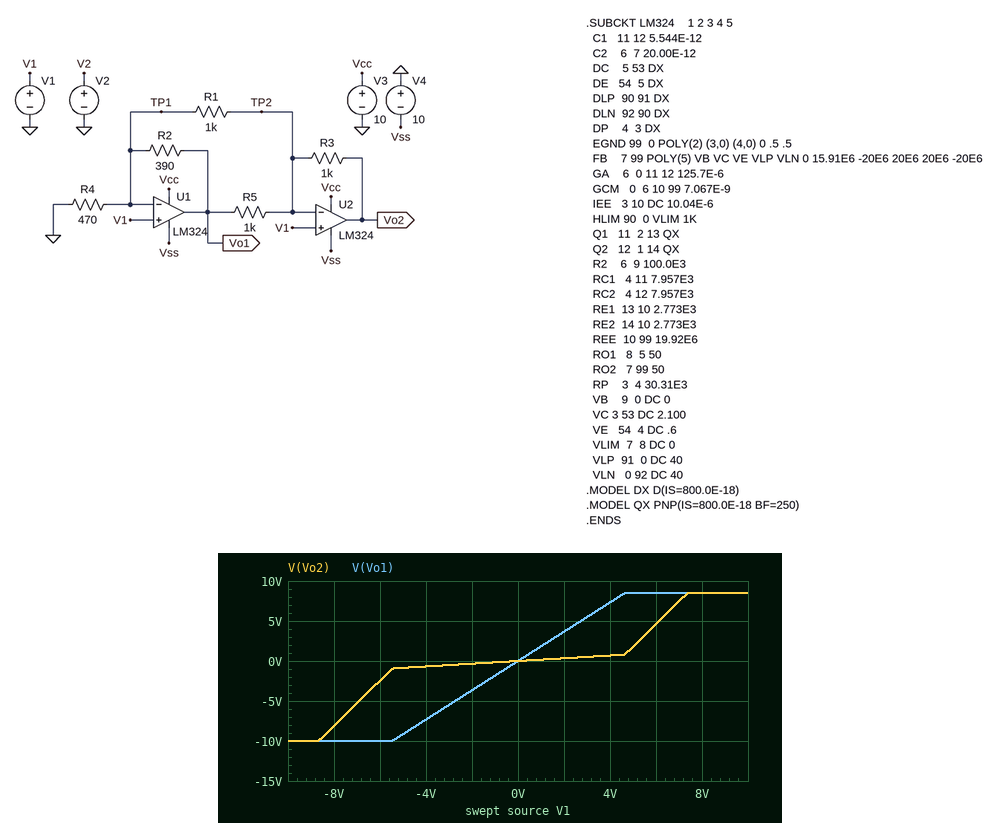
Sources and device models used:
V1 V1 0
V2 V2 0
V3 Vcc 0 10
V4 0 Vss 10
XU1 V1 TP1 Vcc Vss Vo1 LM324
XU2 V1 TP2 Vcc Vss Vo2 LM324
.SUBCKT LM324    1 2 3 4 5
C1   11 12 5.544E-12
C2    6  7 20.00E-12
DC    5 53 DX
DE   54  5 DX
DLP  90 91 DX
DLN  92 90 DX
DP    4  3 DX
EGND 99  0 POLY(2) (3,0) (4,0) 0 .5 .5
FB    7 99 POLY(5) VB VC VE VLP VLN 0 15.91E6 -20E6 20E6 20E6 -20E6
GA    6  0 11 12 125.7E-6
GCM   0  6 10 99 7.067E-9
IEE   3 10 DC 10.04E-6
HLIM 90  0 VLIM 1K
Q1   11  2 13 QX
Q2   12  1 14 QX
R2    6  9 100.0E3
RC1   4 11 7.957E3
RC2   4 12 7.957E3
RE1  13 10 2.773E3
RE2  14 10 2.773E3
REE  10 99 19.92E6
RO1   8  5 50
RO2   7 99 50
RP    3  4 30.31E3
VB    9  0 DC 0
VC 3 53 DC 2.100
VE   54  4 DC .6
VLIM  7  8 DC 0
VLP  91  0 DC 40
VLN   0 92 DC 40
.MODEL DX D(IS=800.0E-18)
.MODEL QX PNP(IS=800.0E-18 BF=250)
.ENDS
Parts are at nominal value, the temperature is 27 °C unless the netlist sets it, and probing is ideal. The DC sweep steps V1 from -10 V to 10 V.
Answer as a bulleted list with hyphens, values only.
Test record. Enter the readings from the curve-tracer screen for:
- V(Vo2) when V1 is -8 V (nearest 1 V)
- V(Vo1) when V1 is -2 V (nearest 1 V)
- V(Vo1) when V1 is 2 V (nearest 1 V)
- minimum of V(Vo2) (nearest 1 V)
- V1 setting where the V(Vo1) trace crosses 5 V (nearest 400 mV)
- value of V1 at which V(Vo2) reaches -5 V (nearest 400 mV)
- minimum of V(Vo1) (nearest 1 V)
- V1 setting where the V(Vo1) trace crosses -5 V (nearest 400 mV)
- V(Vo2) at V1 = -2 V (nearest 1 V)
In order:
- -8 V
- -4 V
- 4 V
- -10 V
- 2.8 V
- -6.8 V
- -10 V
- -2.8 V
- 0 V
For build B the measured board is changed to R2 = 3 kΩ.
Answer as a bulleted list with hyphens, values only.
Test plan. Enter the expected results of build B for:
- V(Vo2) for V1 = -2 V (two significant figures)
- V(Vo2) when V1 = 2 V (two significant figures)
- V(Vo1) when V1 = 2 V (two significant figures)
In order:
- 5.5 V
- -3.9 V
- 8.5 V
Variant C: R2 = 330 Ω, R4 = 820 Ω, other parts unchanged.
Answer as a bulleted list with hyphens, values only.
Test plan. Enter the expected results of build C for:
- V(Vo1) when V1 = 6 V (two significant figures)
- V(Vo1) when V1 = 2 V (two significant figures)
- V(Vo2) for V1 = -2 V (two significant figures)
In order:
- 8.4 V
- 2.8 V
- -1.2 V
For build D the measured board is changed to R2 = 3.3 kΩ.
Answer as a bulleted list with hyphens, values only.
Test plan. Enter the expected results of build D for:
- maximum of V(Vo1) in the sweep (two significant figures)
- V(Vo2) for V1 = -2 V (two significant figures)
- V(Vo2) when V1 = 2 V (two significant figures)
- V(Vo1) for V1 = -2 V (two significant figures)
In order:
- 8.5 V
- 5.5 V
- -3.8 V
- -10 V
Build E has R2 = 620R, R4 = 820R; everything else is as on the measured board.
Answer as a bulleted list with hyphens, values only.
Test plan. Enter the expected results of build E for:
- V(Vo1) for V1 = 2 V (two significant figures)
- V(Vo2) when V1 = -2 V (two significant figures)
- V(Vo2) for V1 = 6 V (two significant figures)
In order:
- 3.5 V
- -490 mV
- 4.4 V
